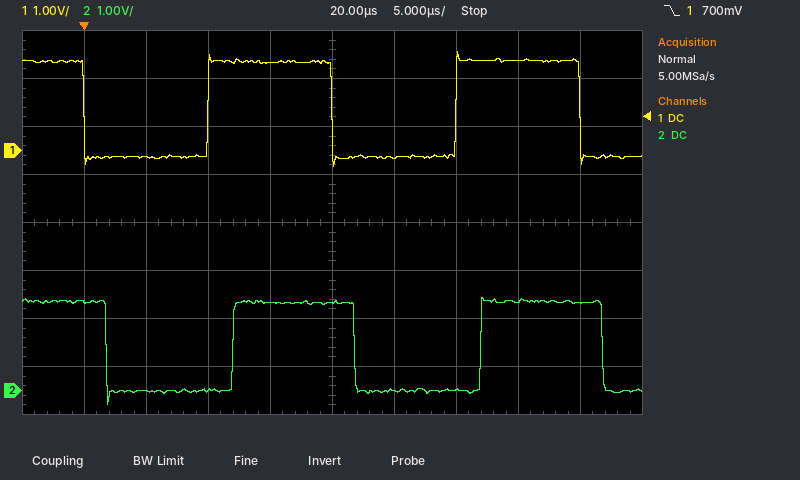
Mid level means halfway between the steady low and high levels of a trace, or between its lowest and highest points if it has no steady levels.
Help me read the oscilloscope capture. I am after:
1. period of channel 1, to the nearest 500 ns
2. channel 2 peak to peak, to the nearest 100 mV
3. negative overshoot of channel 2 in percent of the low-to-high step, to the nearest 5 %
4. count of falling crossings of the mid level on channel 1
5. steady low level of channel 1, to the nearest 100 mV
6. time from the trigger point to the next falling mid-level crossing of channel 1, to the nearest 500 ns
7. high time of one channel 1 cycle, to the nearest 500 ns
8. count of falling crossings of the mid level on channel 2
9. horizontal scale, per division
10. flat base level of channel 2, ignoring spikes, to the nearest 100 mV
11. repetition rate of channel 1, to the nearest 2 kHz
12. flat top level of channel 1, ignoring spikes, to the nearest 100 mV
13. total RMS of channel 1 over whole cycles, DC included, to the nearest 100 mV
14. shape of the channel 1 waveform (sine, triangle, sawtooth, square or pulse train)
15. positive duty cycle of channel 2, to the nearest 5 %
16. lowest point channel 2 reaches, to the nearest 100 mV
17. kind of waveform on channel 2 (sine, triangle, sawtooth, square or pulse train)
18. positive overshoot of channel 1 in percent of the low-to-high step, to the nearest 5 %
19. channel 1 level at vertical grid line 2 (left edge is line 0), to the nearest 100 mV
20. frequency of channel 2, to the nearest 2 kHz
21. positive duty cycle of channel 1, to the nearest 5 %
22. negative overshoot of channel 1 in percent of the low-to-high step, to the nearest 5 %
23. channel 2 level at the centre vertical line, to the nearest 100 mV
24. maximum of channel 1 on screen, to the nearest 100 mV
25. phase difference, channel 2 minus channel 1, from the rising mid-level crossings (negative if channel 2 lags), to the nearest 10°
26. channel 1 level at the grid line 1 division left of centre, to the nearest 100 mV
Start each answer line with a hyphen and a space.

- 20.0 µs
- 2.2 V
- 15 %
- 3
- -100 mV
- 20.0 µs
- 10.0 µs
- 3
- 5 µs
- 0.0 V
- 50 kHz
- 1.9 V
- 1.3 V
- square
- 50 %
- -300 mV
- square
- 10 %
- -100 mV
- 50 kHz
- 50 %
- 10 %
- 1.8 V
- 2.1 V
- -40°
- 1.8 V
